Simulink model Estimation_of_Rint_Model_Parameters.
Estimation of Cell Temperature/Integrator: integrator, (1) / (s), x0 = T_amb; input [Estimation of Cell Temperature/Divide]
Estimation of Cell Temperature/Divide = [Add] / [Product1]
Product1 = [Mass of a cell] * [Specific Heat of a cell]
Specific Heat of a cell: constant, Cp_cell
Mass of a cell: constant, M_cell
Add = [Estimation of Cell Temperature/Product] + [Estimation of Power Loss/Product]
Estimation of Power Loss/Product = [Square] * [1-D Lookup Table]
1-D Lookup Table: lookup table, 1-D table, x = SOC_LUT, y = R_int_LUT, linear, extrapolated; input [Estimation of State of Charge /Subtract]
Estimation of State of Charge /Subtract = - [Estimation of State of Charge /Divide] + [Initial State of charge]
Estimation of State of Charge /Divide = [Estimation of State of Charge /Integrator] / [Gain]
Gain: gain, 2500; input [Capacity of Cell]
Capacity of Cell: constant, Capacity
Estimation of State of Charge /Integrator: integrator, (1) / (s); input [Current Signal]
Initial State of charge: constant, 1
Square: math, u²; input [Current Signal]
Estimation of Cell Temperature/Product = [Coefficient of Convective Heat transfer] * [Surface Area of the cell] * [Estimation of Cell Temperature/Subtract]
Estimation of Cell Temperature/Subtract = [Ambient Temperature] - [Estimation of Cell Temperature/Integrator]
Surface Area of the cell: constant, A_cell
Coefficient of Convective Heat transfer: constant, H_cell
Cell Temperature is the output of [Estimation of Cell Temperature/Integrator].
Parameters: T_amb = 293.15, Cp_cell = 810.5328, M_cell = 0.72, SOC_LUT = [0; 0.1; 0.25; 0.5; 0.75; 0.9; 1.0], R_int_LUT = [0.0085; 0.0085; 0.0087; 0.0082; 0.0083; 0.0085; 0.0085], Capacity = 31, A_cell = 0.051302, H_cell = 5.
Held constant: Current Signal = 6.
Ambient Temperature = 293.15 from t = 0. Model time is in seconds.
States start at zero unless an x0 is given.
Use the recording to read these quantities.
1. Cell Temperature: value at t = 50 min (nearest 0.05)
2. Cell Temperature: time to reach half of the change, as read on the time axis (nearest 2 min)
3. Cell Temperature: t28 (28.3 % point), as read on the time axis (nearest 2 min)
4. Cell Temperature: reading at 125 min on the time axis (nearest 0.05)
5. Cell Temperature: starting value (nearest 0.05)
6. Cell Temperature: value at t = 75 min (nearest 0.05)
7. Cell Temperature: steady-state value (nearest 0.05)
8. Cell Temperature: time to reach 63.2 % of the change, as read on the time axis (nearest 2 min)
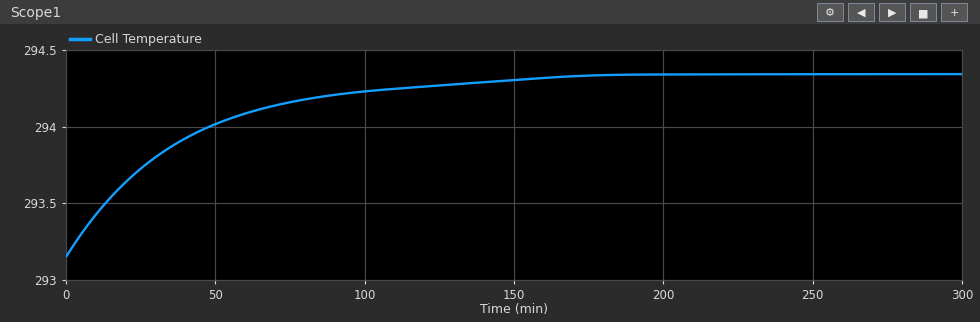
294.00
26 min
12 min
294.25
293.15
294.15
294.35
38 min
